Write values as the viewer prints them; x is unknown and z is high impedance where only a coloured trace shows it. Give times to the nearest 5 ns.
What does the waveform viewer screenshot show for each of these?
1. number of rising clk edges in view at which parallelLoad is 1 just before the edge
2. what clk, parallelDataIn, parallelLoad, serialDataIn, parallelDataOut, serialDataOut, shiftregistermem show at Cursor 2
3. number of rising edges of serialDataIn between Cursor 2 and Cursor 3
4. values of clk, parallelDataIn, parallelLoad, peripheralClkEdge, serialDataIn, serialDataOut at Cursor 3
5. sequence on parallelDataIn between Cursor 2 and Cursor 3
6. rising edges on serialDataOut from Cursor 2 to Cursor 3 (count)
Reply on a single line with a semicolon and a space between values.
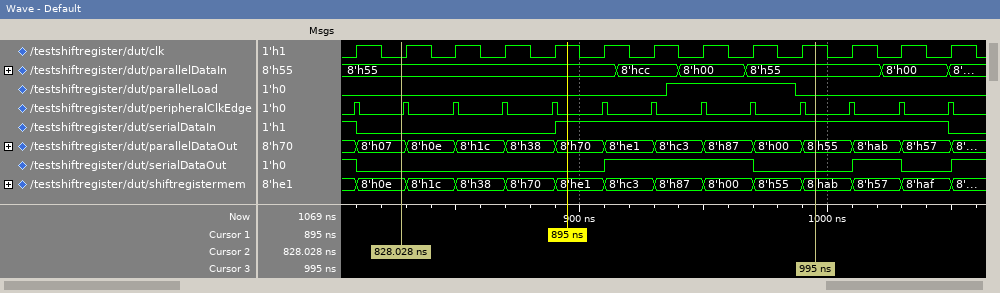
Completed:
2; clk=0, parallelDataIn=8'h55, parallelLoad=0, serialDataIn=0, parallelDataOut=8'h07, serialDataOut=0, shiftregistermem=8'h0e; 1; clk=1, parallelDataIn=8'h55, parallelLoad=0, peripheralClkEdge=0, serialDataIn=1, serialDataOut=0; 8'h55, 8'hcc, 8'h00, 8'h55; 1
